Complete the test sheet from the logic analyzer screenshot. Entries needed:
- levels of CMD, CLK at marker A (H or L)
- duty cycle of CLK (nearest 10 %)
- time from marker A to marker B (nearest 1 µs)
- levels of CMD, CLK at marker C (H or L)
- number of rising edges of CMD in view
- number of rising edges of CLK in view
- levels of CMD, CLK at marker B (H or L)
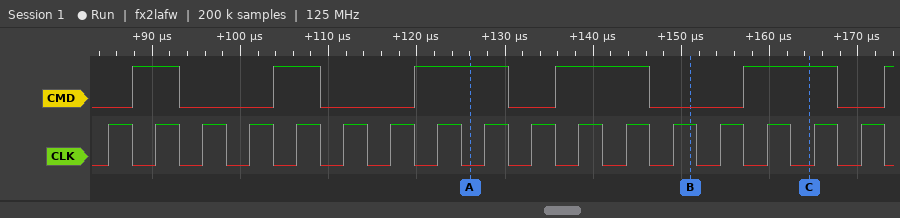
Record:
CMD=H, CLK=L
50 %
25 µs
CMD=H, CLK=L
6
17
CMD=L, CLK=H
